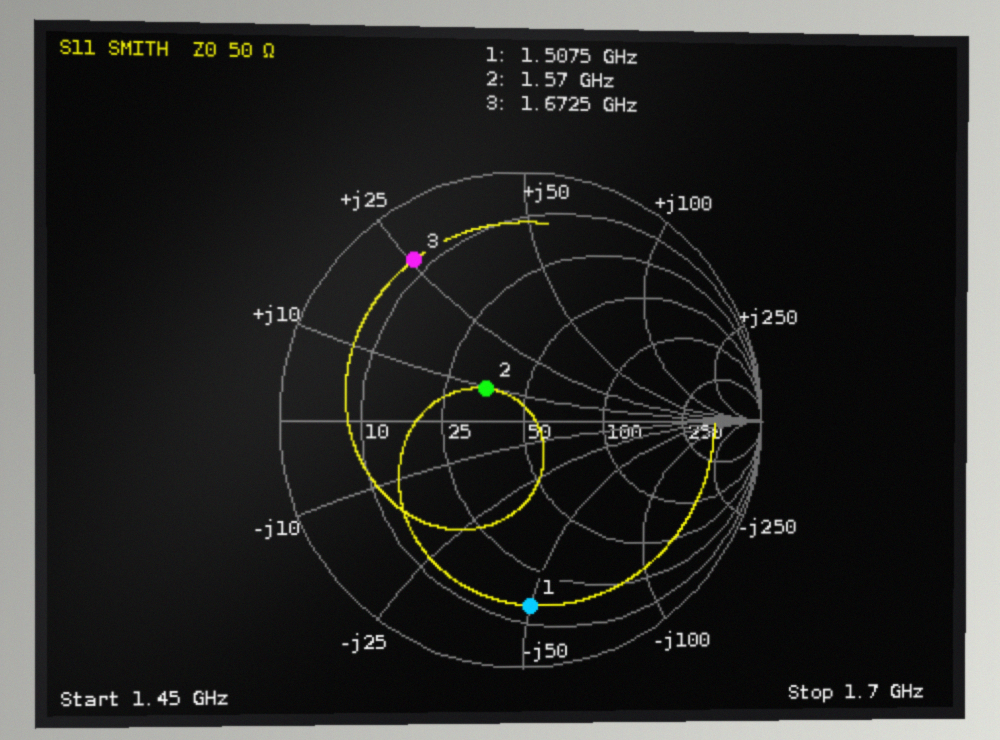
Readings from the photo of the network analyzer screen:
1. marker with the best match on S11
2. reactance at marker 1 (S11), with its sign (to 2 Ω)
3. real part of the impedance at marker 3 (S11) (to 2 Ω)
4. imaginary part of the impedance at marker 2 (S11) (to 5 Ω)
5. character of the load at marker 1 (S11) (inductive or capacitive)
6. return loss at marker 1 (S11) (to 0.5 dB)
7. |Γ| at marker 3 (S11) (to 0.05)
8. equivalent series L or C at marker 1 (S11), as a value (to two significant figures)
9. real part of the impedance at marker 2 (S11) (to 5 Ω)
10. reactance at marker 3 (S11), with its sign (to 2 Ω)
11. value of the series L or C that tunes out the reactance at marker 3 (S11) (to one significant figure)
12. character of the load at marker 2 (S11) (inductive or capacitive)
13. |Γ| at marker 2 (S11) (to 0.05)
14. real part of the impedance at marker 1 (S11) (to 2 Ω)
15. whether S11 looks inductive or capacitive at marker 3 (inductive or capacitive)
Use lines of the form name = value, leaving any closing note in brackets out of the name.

marker with the best match on S11 = marker 2
reactance at marker 1 (S11), with its sign = -50 Ω
real part of the impedance at marker 3 (S11) = 8 Ω
imaginary part of the impedance at marker 2 (S11) = +10 Ω
character of the load at marker 1 (S11) = capacitive
return loss at marker 1 (S11) = 2.5 dB
|Γ| at marker 3 (S11) = 0.80
equivalent series L or C at marker 1 (S11), as a value = 2.1 pF
real part of the impedance at marker 2 (S11) = 35 Ω
reactance at marker 3 (S11), with its sign = +26 Ω
value of the series L or C that tunes out the reactance at marker 3 (S11) = 4 pF
character of the load at marker 2 (S11) = inductive
|Γ| at marker 2 (S11) = 0.20
real part of the impedance at marker 1 (S11) = 14 Ω
whether S11 looks inductive or capacitive at marker 3 = inductive
